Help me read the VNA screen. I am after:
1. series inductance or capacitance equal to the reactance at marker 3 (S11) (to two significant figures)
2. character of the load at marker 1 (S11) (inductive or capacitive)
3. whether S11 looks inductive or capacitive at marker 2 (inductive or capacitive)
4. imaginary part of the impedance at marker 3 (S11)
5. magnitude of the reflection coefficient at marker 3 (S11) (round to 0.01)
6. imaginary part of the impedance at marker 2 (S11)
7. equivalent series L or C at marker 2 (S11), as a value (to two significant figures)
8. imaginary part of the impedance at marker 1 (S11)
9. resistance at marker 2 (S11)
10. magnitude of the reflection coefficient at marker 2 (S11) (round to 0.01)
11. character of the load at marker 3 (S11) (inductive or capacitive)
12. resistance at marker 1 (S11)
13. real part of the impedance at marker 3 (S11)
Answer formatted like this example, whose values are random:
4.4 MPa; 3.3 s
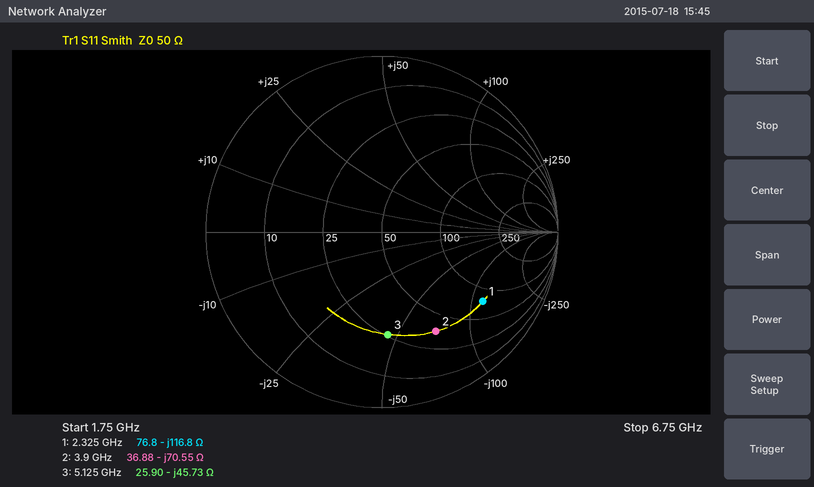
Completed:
680 fF; capacitive; capacitive; -45.73 Ω; 0.58; -70.55 Ω; 580 fF; -116.8 Ω; 36.88 Ω; 0.64; capacitive; 76.8 Ω; 25.90 Ω
